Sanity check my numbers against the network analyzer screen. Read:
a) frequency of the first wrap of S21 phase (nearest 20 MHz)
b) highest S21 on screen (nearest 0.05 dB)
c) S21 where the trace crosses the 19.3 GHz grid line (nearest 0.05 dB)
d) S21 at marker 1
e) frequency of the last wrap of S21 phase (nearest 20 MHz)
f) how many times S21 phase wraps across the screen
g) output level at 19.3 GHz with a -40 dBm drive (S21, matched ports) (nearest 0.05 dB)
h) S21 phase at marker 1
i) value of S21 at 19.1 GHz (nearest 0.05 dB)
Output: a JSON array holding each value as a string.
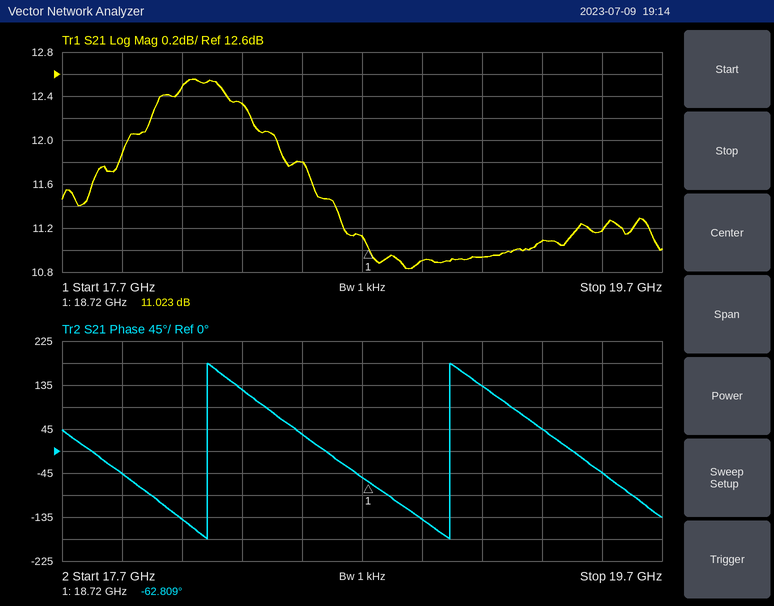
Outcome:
["18.18 GHz", "12.55 dB", "11.10 dB", "11.023 dB", "19.00 GHz", "2", "-28.90 dBm", "-62.809°", "10.95 dB"]
